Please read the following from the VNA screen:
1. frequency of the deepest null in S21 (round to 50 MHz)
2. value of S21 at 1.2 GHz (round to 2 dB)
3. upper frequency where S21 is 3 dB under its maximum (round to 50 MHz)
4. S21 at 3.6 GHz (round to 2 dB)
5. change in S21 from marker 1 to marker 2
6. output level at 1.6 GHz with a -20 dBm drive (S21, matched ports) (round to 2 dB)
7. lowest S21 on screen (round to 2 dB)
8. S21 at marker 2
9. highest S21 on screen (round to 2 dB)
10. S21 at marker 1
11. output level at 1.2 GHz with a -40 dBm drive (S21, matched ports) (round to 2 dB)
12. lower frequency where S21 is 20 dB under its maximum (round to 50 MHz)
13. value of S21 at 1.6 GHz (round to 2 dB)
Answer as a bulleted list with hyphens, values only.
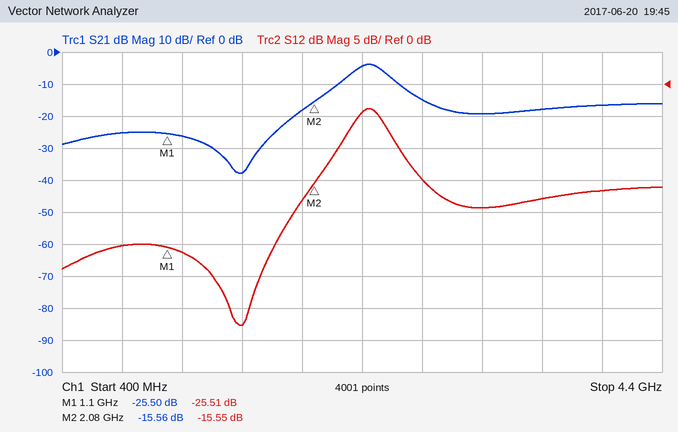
- 1.60 GHz
- -26 dB
- 2.55 GHz
- -18 dB
- 9.94 dB
- -58 dBm
- -38 dB
- -15.56 dB
- -4 dB
- -25.50 dB
- -66 dBm
- 1.85 GHz
- -38 dB
